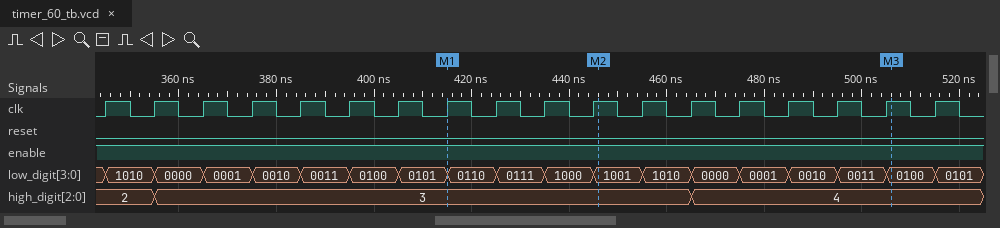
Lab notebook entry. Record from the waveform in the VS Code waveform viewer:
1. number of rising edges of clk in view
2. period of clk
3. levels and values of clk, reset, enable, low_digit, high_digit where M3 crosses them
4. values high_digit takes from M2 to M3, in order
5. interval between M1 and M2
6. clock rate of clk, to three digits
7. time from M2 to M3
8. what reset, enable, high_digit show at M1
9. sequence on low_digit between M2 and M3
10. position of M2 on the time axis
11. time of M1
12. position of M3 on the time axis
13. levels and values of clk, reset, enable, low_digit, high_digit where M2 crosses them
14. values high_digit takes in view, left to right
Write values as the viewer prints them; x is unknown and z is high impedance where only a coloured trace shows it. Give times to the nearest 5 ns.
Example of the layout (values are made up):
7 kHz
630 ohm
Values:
18
10 ns
clk=1, reset=0, enable=1, low_digit=0100, high_digit=4
3, 4
30 ns
100 MHz
60 ns
reset=0, enable=1, high_digit=3
1001, 1010, 0000, 0001, 0010, 0011, 0100
445 ns
415 ns
505 ns
clk=1, reset=0, enable=1, low_digit=1001, high_digit=3
2, 3, 4
